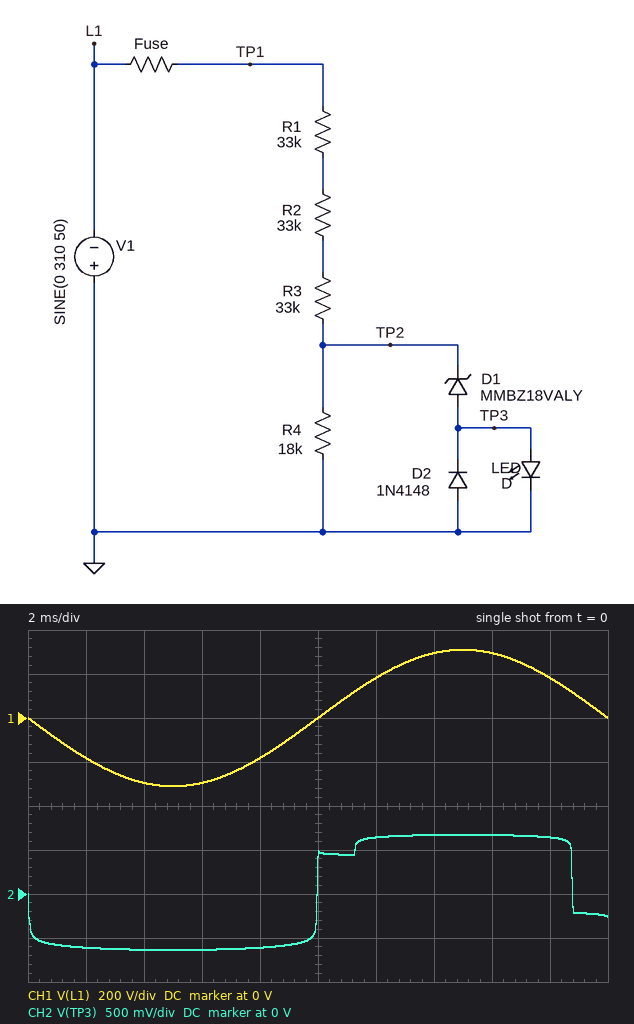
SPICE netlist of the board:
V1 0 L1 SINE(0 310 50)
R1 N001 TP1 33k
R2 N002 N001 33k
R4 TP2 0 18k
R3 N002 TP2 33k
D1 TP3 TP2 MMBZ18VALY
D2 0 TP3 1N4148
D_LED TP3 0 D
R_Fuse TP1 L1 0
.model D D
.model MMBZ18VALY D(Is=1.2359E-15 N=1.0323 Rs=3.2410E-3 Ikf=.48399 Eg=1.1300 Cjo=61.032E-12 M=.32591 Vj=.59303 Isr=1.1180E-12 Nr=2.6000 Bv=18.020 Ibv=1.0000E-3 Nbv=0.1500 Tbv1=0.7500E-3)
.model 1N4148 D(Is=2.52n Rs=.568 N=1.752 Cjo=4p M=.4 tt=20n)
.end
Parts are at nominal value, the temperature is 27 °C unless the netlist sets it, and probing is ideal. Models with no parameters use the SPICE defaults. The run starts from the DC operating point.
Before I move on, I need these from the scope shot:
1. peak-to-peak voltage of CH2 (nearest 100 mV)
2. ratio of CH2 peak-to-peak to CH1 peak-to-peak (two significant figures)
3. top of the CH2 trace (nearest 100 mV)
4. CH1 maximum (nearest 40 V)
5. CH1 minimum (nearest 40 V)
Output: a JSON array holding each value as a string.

["1.3 V", "0.0021", "700 mV", "320 V", "-320 V"]
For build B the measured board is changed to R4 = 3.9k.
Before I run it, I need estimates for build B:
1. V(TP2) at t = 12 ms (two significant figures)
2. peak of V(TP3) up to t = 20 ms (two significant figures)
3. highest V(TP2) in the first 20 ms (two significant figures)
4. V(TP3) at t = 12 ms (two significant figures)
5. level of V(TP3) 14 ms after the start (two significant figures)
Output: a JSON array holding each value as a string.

["6.9 V", "440 mV", "12 V", "410 mV", "380 mV"]
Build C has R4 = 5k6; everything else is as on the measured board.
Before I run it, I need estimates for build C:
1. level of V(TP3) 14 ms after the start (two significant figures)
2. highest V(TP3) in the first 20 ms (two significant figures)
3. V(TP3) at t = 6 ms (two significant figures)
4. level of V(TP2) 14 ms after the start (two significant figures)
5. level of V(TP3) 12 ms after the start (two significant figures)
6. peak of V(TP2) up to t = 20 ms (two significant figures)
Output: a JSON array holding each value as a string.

["390 mV", "450 mV", "-630 mV", "16 V", "420 mV", "17 V"]
